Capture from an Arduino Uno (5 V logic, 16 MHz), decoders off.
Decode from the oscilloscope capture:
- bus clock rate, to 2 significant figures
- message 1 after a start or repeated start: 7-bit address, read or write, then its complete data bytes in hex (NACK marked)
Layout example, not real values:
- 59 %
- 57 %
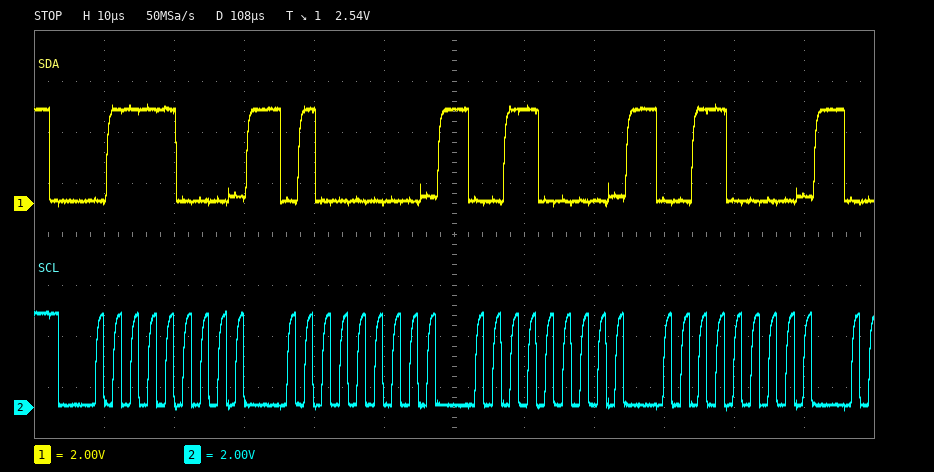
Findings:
- 400 kHz
- 0x3C write: 40 30 30
